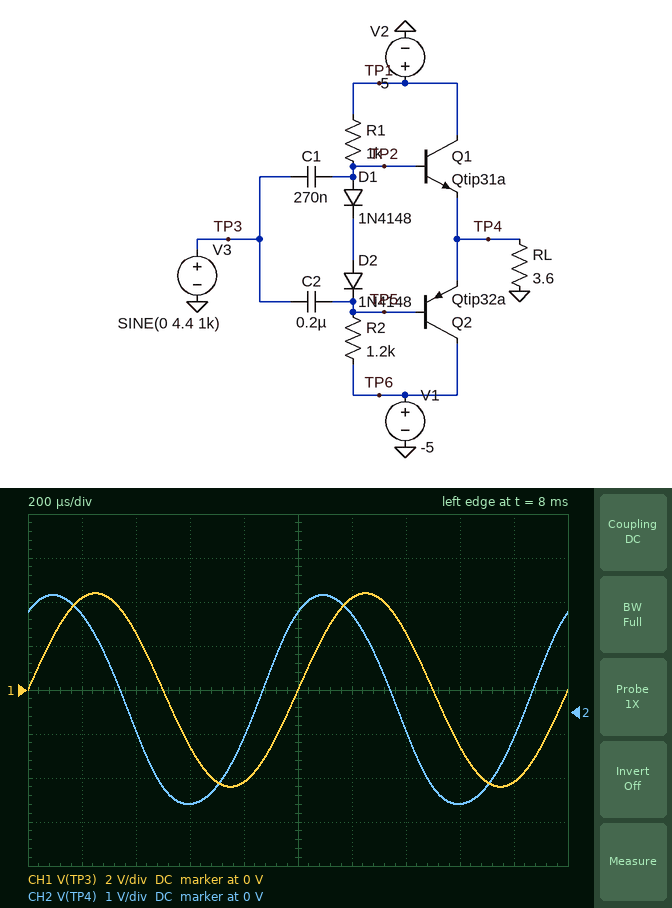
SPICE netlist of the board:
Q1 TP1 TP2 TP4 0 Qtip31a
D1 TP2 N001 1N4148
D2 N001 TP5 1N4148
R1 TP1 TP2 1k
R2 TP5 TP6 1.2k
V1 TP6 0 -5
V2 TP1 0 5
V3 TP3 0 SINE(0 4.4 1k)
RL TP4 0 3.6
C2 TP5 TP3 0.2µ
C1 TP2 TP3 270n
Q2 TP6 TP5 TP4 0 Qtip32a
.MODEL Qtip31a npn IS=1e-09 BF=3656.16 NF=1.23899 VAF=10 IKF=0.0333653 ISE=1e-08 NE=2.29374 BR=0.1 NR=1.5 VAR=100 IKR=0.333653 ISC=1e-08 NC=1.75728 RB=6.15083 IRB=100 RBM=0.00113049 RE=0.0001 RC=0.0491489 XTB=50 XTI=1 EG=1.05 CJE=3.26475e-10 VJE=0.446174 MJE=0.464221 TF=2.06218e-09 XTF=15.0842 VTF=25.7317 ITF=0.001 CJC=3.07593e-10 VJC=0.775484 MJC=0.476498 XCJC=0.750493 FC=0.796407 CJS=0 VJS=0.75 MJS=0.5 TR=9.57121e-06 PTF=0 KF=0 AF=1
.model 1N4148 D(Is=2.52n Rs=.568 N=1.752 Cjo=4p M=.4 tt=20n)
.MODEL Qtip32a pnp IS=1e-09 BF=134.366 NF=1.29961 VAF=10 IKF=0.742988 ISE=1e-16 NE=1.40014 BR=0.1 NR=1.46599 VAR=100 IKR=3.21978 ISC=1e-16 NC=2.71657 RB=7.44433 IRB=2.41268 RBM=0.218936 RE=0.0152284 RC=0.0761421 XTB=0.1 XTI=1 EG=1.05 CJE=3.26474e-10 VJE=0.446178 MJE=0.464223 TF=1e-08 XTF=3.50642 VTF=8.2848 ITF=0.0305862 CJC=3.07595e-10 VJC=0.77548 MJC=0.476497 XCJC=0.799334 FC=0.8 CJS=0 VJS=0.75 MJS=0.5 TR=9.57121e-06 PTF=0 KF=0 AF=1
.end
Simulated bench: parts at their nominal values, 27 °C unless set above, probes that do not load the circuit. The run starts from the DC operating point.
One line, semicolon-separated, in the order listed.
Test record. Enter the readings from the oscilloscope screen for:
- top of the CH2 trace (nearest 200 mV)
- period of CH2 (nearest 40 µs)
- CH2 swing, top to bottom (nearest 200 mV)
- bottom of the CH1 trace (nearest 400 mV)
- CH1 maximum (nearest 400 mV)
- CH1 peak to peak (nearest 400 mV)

2.6 V; 1.00 ms; 4.8 V; -4.4 V; 4.4 V; 8.8 V
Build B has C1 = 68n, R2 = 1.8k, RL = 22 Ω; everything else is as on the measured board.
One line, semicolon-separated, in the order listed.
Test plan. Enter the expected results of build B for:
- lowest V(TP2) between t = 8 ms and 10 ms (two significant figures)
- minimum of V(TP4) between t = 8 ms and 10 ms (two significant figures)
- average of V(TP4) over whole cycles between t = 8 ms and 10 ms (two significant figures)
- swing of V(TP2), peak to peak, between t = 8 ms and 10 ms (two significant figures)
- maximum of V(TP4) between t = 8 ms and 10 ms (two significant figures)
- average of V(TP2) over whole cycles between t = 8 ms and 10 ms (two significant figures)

-1.0 V; -1.6 V; 1.2 V; 5.7 V; 4.0 V; 1.8 V
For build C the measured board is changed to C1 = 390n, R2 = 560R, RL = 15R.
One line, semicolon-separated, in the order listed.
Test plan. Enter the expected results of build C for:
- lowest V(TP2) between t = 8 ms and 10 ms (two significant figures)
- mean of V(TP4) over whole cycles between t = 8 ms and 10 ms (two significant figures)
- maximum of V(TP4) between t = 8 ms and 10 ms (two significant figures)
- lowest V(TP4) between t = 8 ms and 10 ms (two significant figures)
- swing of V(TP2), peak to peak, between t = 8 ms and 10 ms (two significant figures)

-3.6 V; -890 mV; 2.3 V; -4.1 V; 6.6 V
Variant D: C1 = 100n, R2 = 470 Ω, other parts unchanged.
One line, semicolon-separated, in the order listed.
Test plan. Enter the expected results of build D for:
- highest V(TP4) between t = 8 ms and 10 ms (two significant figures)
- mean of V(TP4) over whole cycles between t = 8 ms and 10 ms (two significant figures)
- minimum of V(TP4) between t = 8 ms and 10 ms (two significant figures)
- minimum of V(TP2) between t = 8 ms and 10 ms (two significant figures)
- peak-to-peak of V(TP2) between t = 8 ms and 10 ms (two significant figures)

640 mV; -760 mV; -2.1 V; -1.5 V; 2.9 V
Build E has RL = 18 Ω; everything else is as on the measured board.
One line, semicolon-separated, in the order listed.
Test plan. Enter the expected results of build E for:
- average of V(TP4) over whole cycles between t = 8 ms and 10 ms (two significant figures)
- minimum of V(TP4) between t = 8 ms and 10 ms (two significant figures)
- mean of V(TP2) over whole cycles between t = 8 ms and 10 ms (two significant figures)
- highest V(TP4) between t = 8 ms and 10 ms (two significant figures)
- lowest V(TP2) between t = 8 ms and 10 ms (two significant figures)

450 mV; -3.0 V; 1.1 V; 3.9 V; -2.4 V
